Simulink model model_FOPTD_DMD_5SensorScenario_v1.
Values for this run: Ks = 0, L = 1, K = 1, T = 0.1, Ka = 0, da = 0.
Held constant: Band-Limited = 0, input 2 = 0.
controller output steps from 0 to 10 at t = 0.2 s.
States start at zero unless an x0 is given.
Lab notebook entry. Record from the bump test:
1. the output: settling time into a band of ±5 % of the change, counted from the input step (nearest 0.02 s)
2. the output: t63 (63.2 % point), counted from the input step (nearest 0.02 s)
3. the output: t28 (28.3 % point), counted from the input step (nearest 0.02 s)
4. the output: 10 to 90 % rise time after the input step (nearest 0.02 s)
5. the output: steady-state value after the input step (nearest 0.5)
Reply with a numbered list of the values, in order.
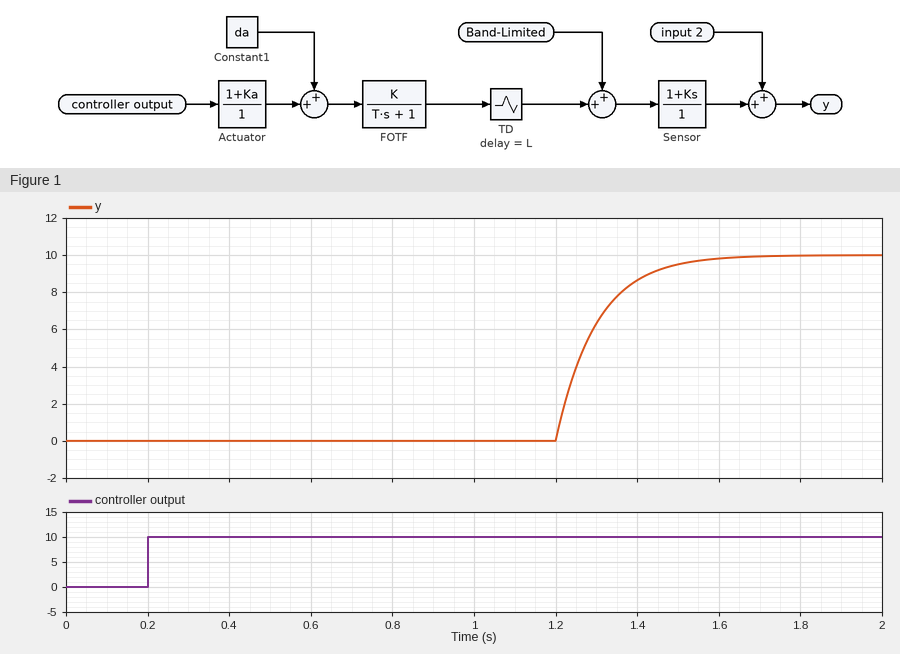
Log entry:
1. 1.30 s
2. 1.10 s
3. 1.04 s
4. 0.22 s
5. 10.0
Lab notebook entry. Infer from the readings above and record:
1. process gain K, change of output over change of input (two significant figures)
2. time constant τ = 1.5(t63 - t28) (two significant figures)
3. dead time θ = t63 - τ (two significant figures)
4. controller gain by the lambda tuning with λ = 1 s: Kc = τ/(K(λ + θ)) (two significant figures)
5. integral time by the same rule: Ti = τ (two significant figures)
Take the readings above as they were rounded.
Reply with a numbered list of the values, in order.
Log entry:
1. 1.0
2. 0.090 s
3. 1.0 s
4. 0.045
5. 0.090 s
